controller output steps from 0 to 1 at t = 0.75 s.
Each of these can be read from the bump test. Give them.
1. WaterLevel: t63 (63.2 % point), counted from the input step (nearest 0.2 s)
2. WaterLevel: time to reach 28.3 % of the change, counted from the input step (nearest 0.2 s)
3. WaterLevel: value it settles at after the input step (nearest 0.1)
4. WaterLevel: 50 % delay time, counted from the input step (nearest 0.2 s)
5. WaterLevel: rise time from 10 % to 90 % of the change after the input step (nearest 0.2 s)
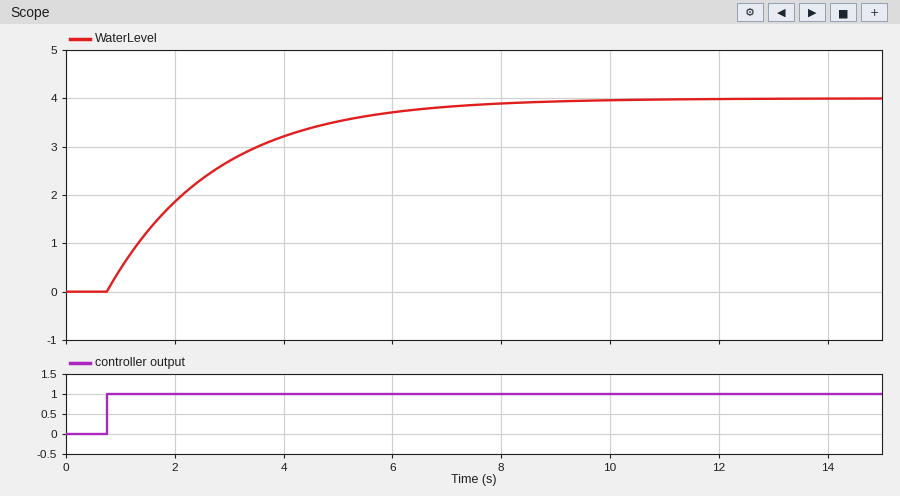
2.0 s
0.6 s
4.0
1.4 s
4.4 s
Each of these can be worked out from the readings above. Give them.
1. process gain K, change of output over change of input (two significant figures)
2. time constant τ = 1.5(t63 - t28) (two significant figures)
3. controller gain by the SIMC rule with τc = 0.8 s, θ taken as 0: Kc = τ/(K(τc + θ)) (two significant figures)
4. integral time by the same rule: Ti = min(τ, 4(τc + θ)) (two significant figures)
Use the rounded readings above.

4.0
2.1 s
0.66
2.1 s
